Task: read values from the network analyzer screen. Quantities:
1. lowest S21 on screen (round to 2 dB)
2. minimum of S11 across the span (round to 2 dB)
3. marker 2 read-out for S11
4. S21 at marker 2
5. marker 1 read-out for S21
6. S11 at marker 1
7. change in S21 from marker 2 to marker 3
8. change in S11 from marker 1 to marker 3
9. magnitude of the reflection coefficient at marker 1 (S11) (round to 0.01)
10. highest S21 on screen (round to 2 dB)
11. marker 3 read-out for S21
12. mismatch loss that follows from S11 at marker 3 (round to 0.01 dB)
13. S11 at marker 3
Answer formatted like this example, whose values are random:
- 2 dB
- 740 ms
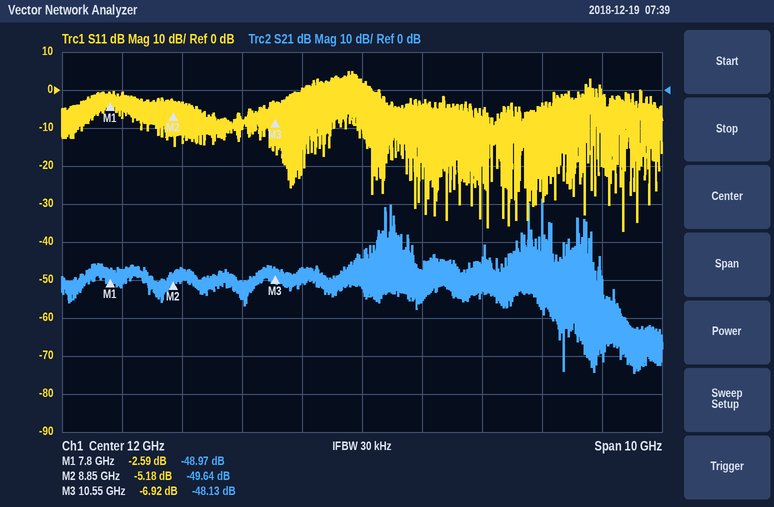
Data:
- -74 dB
- -38 dB
- -5.18 dB
- -49.64 dB
- -48.97 dB
- -2.59 dB
- 1.51 dB
- -4.33 dB
- 0.74
- -28 dB
- -48.13 dB
- 0.99 dB
- -6.92 dB
